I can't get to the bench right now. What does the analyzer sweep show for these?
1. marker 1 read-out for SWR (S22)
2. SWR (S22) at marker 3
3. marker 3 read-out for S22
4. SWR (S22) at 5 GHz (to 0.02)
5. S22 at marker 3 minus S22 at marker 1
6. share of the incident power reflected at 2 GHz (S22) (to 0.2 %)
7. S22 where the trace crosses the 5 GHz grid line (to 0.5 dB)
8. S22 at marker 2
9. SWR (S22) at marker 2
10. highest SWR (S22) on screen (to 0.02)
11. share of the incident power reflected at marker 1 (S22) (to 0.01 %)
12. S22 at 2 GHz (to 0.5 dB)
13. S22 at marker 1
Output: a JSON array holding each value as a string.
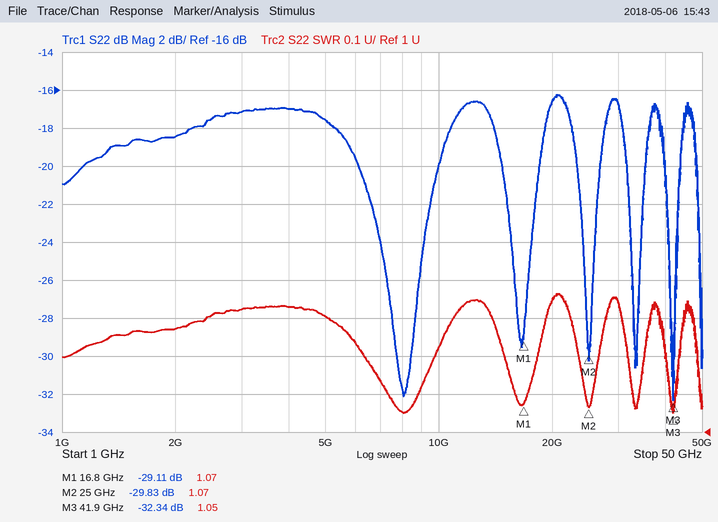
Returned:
["1.07", "1.05", "-32.34 dB", "1.30", "-3.23 dB", "1.4 %", "-17.5 dB", "-29.83 dB", "1.07", "1.36", "0.12 %", "-18.5 dB", "-29.11 dB"]
